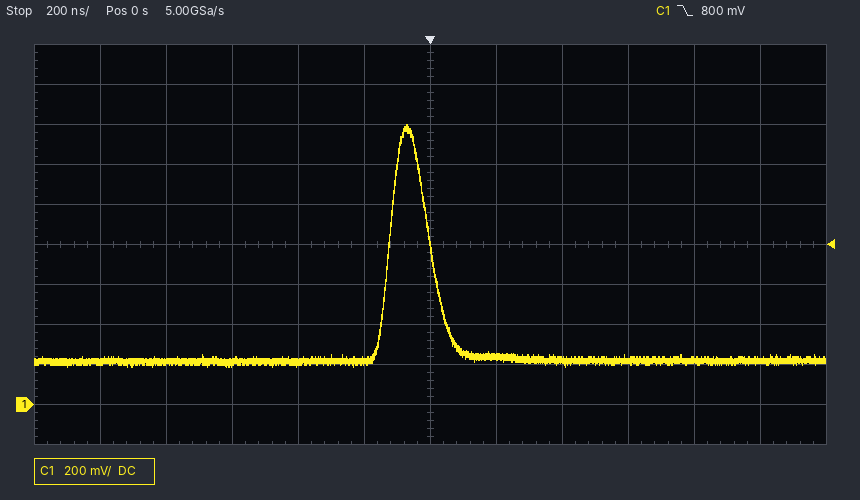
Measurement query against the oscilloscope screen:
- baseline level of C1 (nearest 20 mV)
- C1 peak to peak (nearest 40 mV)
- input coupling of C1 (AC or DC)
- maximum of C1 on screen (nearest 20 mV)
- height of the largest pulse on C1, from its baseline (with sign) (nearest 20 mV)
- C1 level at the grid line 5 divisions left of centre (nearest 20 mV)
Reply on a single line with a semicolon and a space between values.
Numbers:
220 mV; 1.20 V; DC; 1.40 V; +1.18 V; 220 mV
